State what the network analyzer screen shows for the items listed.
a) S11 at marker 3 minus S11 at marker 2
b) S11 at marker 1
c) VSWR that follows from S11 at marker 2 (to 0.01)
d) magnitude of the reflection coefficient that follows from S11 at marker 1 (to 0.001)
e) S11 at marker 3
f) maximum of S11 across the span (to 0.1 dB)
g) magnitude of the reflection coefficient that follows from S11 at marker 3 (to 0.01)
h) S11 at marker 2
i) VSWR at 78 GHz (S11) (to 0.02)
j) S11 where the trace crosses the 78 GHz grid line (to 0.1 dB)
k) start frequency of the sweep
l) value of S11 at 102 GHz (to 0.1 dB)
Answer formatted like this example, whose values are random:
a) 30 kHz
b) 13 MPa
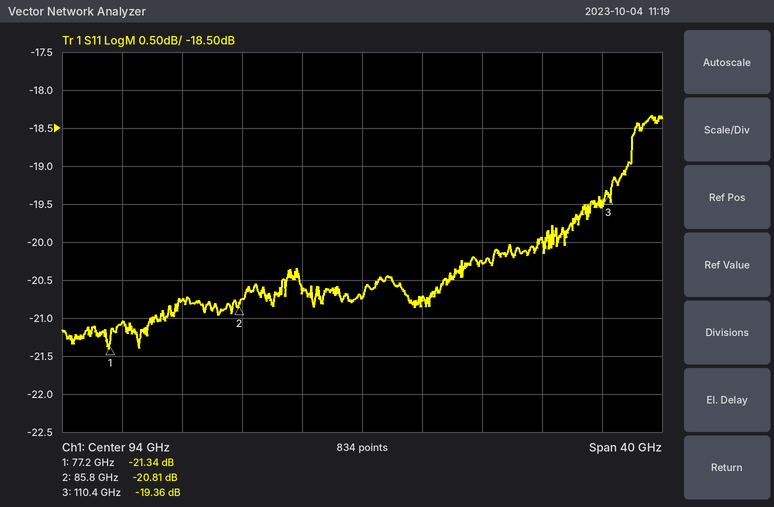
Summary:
a) 1.45 dB
b) -21.34 dB
c) 1.20
d) 0.086
e) -19.36 dB
f) -18.3 dB
g) 0.11
h) -20.81 dB
i) 1.20
j) -21.1 dB
k) 74 GHz
l) -20.3 dB
